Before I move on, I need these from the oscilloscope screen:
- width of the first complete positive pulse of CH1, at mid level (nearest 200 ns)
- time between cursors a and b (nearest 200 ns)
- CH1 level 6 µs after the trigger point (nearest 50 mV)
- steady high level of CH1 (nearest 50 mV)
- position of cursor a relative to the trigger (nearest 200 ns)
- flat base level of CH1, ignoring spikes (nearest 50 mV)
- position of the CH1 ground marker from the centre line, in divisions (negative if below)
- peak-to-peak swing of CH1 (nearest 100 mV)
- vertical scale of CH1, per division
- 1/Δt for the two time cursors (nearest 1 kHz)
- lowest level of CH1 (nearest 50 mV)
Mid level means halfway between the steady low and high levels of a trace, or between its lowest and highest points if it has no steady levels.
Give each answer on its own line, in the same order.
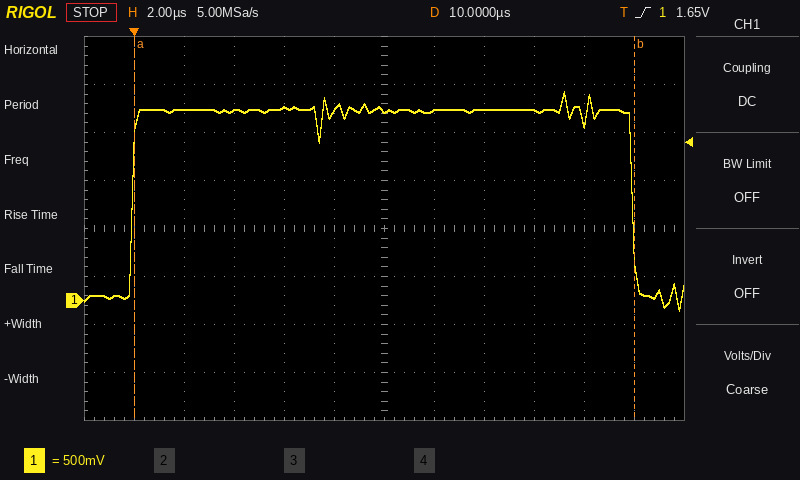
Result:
20.0 µs
20.0 µs
2.00 V
2.00 V
0.0 µs
50 mV
-1.5 div
2.30 V
500 mV
50 kHz
-100 mV
